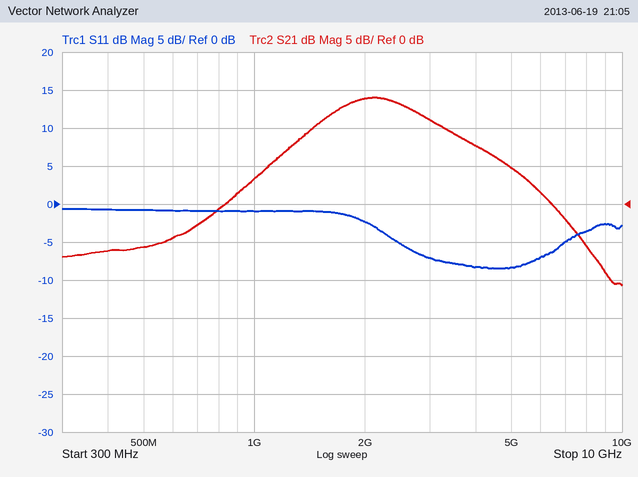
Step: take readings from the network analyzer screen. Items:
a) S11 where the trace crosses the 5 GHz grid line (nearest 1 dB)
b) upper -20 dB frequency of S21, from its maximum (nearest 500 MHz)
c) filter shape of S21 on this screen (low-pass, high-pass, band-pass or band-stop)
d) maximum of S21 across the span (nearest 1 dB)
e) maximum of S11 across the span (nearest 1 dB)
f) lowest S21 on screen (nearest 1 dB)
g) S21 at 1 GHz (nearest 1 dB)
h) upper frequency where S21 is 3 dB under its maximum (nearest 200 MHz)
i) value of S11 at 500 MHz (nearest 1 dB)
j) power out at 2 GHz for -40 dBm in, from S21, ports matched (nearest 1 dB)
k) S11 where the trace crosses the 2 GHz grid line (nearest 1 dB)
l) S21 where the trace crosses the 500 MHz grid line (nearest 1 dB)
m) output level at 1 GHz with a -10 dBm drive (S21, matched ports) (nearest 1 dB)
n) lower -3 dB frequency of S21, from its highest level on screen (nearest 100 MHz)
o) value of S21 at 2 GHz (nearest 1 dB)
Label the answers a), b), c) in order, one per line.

a) -8 dB
b) 8.0 GHz
c) band-pass
d) 14 dB
e) -1 dB
f) -11 dB
g) 3 dB
h) 3.0 GHz
i) -1 dB
j) -26 dBm
k) -2 dB
l) -6 dB
m) -7 dBm
n) 1.5 GHz
o) 14 dB
